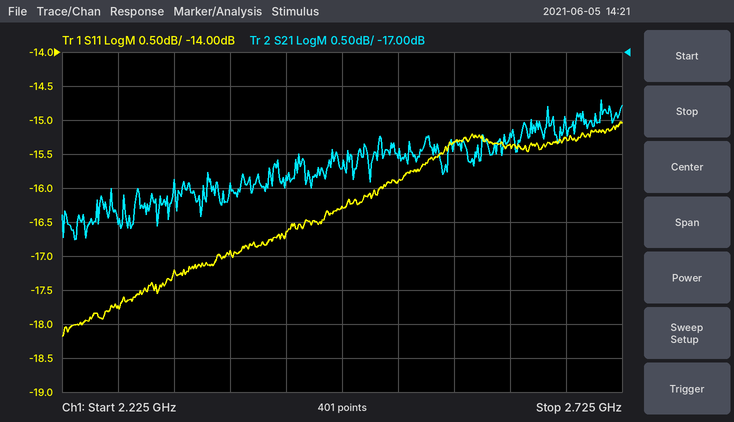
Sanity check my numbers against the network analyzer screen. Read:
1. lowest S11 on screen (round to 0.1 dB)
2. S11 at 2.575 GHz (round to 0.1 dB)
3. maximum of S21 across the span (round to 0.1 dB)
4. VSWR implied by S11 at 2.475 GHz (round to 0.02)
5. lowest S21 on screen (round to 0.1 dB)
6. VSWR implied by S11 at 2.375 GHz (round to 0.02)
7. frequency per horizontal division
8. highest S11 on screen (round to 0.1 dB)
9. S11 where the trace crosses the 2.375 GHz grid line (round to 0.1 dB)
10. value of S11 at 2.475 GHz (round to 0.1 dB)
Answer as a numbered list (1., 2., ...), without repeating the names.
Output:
1. -18.2 dB
2. -15.3 dB
3. -17.7 dB
4. 1.36
5. -19.8 dB
6. 1.34
7. 50 MHz
8. -15.0 dB
9. -16.9 dB
10. -16.3 dB
